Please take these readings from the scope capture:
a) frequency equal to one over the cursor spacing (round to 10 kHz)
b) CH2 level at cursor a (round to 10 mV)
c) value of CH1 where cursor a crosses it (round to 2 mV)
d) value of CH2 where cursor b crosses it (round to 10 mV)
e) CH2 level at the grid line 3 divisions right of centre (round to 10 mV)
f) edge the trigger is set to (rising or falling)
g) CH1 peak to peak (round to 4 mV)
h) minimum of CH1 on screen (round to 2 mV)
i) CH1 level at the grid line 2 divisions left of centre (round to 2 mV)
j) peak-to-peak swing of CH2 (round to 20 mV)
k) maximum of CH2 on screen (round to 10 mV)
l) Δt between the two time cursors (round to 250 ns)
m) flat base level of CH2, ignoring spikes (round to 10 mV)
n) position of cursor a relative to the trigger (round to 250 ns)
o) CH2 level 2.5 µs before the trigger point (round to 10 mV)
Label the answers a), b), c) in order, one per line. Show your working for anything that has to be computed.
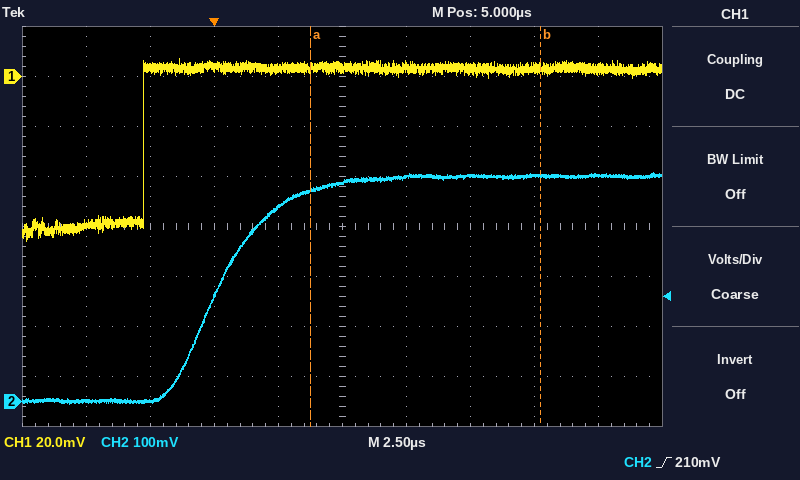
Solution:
a) 1 / 9.00 µs ≈ 110 kHz
b) 420 mV
c) 4 mV
d) 450 mV
e) 450 mV
f) rising
g) 72 mV
h) -66 mV
i) 4 mV
j) 460 mV
k) 460 mV
l) 9.00 µs
m) 0 mV
n) +3.75 µs
o) 0 mV
